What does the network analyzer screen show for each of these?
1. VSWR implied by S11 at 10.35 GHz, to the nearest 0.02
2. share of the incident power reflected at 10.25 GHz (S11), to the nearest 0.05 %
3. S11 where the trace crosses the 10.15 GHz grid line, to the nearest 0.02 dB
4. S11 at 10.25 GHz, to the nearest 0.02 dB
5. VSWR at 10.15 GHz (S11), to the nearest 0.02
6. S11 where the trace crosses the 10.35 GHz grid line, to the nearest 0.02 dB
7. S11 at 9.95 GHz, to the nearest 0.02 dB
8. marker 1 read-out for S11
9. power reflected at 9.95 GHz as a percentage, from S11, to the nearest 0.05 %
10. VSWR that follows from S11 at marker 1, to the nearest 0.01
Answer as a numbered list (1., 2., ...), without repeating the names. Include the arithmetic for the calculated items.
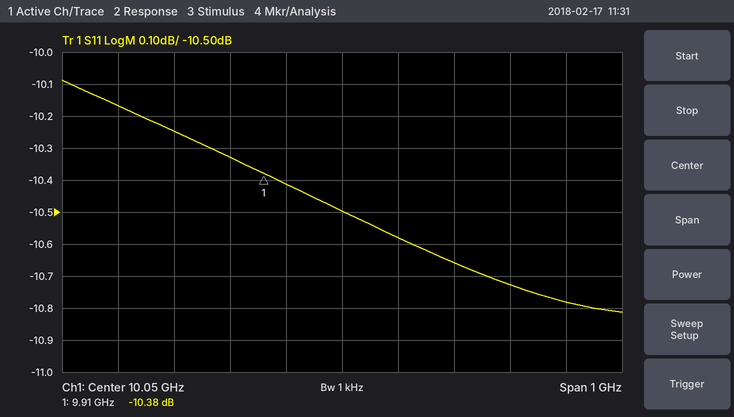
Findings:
1. |Γ| = 10^(-10.72/20) = 0.2911; VSWR = (1 + 0.2911)/(1 − 0.2911) ≈ 1.82
2. 10^(-10.66/10) ≈ 8.59 %, so 8.60 % to the nearest 0.05 %
3. -10.58 dB
4. -10.66 dB
5. |Γ| = 10^(-10.58/20) = 0.2958; VSWR = (1 + 0.2958)/(1 − 0.2958) ≈ 1.84
6. -10.72 dB
7. -10.42 dB
8. -10.38 dB
9. 10^(-10.42/10) ≈ 9.08 %, so 9.10 % to the nearest 0.05 %
10. (1 + 0.3027)/(1 − 0.3027) ≈ 1.87
